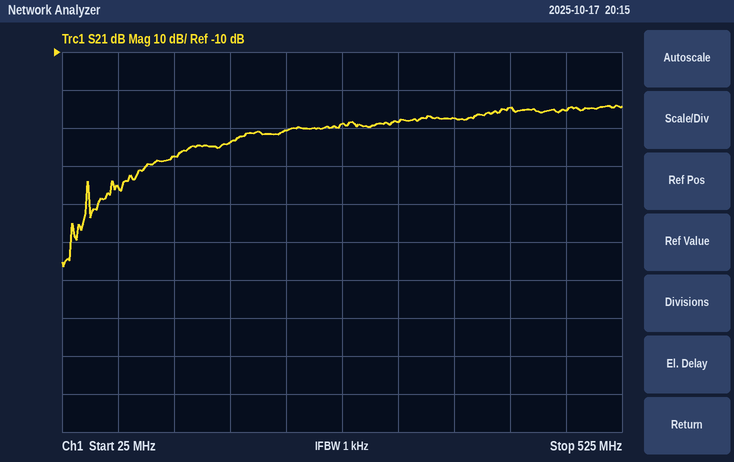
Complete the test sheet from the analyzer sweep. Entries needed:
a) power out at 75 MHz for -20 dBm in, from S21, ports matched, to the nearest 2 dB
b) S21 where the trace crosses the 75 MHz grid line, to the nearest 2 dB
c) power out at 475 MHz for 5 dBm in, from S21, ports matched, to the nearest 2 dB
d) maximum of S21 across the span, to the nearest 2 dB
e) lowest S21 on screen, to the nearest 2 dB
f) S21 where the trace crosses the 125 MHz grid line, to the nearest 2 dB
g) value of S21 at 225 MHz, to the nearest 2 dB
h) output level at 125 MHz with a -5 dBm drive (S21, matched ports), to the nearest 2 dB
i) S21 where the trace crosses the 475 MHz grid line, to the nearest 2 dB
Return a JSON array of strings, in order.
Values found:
["-66 dBm", "-46 dB", "-20 dBm", "-24 dB", "-66 dB", "-38 dB", "-30 dB", "-42 dBm", "-26 dB"]
